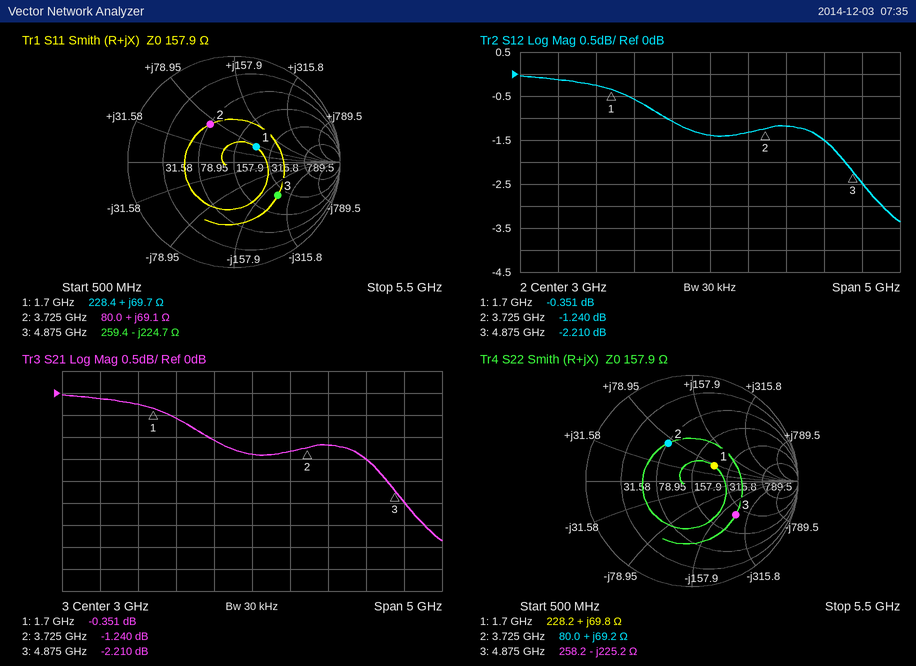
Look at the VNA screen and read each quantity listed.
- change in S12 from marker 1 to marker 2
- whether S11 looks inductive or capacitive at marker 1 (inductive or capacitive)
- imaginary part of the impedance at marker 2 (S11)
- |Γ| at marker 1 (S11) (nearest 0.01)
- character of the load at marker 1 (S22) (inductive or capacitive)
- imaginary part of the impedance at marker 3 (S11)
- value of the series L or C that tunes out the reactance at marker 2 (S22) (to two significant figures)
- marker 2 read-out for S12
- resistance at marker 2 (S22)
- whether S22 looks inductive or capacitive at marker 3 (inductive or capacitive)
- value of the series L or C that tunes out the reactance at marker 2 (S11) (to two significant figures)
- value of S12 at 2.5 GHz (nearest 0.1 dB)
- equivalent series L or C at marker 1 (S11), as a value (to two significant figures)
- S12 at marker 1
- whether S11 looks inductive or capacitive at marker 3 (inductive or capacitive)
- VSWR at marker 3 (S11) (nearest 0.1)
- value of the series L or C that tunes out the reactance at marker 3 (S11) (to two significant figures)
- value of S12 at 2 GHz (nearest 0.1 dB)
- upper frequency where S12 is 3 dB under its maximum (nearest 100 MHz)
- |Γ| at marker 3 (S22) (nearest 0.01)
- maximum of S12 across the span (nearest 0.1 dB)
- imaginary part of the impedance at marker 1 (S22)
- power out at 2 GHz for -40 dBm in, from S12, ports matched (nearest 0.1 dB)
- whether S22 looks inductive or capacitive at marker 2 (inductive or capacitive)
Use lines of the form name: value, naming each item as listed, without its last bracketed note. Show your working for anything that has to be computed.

change in S12 from marker 1 to marker 2: -1.24 − (-0.351) = -0.889 dB
whether S11 looks inductive or capacitive at marker 1: inductive
imaginary part of the impedance at marker 2: +69.1 Ω
|Γ| at marker 1 (S11): 0.25
character of the load at marker 1 (S22): inductive
imaginary part of the impedance at marker 3: -224.7 Ω
value of the series L or C that tunes out the reactance at marker 2 (S22): C = 1/(2π × 3.725 GHz × 69.2 Ω) ≈ 617 fF, so 620 fF to two significant figures
marker 2 read-out for S12: -1.240 dB
resistance at marker 2: 80.0 Ω
whether S22 looks inductive or capacitive at marker 3: capacitive
value of the series L or C that tunes out the reactance at marker 2 (S11): C = 1/(2π × 3.725 GHz × 69.1 Ω) ≈ 618 fF, so 620 fF to two significant figures
value of S12 at 2.5 GHz: -1.1 dB
equivalent series L or C at marker 1 (S11), as a value: L = 69.7 Ω/(2π × 1.7 GHz) ≈ 6.5 nH
S12 at marker 1: -0.351 dB
whether S11 looks inductive or capacitive at marker 3: capacitive
VSWR at marker 3 (S11): 3.2
value of the series L or C that tunes out the reactance at marker 3 (S11): L = 224.7 Ω/(2π × 4.875 GHz) ≈ 7.3 nH
value of S12 at 2 GHz: -0.6 dB
upper frequency where S12 is 3 dB under its maximum: 5.3 GHz
|Γ| at marker 3 (S22): 0.52
maximum of S12 across the span: 0.0 dB
imaginary part of the impedance at marker 1: +69.8 Ω
power out at 2 GHz for -40 dBm in, from S12, ports matched: -40 dBm + (-0.6 dB) = -40.6 dBm
whether S22 looks inductive or capacitive at marker 2: inductive
